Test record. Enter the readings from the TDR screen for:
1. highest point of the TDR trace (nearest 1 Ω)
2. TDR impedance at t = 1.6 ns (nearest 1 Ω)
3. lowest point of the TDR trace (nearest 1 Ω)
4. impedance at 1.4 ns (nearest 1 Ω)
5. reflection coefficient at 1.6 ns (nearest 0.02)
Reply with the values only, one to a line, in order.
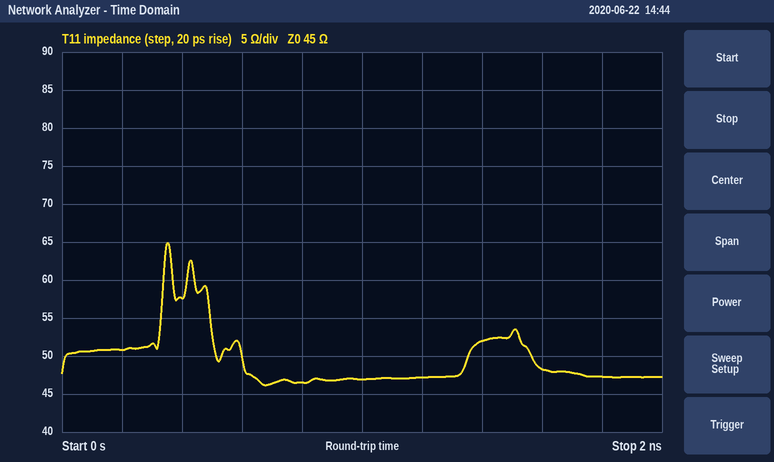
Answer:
65 Ω
48 Ω
46 Ω
52 Ω
+0.04
